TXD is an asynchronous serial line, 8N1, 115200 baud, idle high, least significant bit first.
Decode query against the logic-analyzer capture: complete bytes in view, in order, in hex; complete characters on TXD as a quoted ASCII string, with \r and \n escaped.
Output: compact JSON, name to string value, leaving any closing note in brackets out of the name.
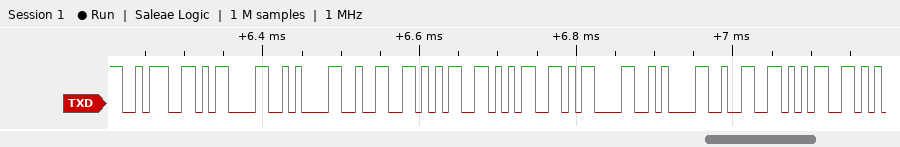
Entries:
{"complete bytes in view, in order, in hex": "0x3A 0x0D 0x0A 0x32 0x35 0x35 0x0D 0x0A 0x32 0x35", "complete characters on TXD as a quoted ASCII string, with \\r and \\n escaped": "\":\\r\\n255\\r\\n25\""}
